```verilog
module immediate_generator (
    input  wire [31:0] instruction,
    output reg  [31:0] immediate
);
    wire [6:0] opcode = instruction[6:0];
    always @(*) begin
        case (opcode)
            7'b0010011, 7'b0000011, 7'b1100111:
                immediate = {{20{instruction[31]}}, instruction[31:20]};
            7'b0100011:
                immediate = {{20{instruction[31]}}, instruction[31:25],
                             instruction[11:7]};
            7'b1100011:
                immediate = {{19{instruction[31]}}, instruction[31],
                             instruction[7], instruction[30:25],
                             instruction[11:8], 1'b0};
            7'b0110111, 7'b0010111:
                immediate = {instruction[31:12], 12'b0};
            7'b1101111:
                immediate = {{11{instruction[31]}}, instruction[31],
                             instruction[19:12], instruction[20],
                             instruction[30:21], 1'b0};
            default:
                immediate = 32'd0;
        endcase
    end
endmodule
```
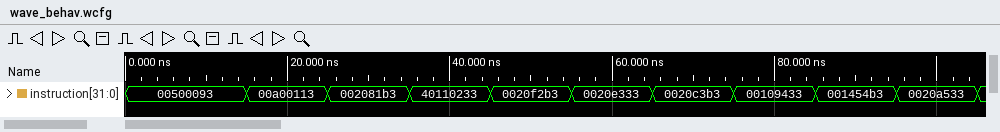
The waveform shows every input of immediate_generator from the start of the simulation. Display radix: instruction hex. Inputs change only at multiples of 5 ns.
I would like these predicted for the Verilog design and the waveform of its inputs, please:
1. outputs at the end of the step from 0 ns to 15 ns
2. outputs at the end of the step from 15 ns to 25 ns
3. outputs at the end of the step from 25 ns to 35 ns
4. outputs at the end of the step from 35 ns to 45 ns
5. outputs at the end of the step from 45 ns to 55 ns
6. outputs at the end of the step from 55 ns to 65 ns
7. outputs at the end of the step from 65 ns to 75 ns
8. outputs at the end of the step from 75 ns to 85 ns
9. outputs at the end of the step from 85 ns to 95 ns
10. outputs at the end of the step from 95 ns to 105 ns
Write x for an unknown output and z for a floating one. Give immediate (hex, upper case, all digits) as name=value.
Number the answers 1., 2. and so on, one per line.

1. immediate=00000005
2. immediate=0000000A
3. immediate=00000000
4. immediate=00000000
5. immediate=00000000
6. immediate=00000000
7. immediate=00000000
8. immediate=00000000
9. immediate=00000000
10. immediate=00000000
